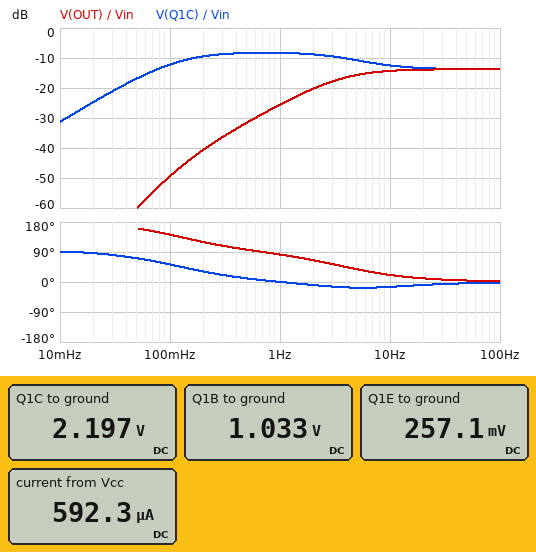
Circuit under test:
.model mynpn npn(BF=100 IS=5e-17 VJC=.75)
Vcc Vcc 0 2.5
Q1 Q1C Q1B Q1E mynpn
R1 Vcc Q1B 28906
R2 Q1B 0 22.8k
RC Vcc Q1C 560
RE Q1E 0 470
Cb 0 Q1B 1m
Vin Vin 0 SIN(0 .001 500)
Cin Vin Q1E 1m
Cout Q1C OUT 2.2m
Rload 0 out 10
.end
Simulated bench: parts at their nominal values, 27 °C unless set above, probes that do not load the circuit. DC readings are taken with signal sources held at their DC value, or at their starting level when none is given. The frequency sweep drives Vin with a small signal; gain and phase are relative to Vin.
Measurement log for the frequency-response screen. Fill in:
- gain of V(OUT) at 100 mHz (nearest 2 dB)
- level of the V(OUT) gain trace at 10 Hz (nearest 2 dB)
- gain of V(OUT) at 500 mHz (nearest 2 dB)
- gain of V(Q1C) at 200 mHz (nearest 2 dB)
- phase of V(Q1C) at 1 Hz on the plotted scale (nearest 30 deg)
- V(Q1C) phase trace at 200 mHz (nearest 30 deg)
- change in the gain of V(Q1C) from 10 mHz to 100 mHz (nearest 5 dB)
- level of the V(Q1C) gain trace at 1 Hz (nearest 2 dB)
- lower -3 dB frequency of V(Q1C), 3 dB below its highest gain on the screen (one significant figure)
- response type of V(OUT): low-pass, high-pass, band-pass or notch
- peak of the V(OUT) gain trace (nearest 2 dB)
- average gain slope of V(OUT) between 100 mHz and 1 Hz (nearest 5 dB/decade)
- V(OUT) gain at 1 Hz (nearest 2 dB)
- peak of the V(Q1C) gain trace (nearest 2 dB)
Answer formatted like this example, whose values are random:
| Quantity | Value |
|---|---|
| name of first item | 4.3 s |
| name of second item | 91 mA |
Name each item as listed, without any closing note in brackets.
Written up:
| Quantity | Value |
|---|---|
| gain of V(OUT) at 100 mHz | -50 dB |
| level of the V(OUT) gain trace at 10 Hz | -14 dB |
| gain of V(OUT) at 500 mHz | -32 dB |
| gain of V(Q1C) at 200 mHz | -10 dB |
| phase of V(Q1C) at 1 Hz on the plotted scale | 0 deg |
| V(Q1C) phase trace at 200 mHz | 30 deg |
| change in the gain of V(Q1C) from 10 mHz to 100 mHz | 20 dB |
| level of the V(Q1C) gain trace at 1 Hz | -8 dB |
| lower -3 dB frequency of V(Q1C), 3 dB below its highest gain on the screen | 100 mHz |
| response type of V(OUT): low-pass, high-pass, band-pass or notch | high-pass |
| peak of the V(OUT) gain trace | -14 dB |
| average gain slope of V(OUT) between 100 mHz and 1 Hz | 25 dB/decade |
| V(OUT) gain at 1 Hz | -26 dB |
| peak of the V(Q1C) gain trace | -8 dB |
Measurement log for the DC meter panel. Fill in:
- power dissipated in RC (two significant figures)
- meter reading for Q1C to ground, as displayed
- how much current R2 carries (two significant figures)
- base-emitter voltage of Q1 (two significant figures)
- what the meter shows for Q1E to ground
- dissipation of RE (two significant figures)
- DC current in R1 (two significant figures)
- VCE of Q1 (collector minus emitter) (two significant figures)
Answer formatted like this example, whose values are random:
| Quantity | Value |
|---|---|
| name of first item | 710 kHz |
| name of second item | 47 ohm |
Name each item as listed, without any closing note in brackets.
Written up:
| Quantity | Value |
|---|---|
| power dissipated in RC | 160 µW |
| meter reading for Q1C to ground, as displayed | 2.197 V |
| how much current R2 carries | 45 µA |
| base-emitter voltage of Q1 | 780 mV |
| what the meter shows for Q1E to ground | 257.1 mV |
| dissipation of RE | 140 µW |
| DC current in R1 | 51 µA |
| VCE of Q1 (collector minus emitter) | 1.9 V |
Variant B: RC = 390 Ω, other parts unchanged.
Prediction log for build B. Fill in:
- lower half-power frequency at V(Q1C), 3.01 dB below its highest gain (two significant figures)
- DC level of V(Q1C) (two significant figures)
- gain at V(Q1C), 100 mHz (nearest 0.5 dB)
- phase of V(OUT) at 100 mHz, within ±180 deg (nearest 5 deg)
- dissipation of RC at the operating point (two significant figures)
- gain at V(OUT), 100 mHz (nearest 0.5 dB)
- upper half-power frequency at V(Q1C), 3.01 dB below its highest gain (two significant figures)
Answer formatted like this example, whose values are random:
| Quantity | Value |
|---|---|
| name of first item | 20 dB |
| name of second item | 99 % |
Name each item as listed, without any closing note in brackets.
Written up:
| Quantity | Value |
|---|---|
| lower half-power frequency at V(Q1C), 3.01 dB below its highest gain | 170 mHz |
| DC level of V(Q1C) | 2.3 V |
| gain at V(Q1C), 100 mHz | -14.5 dB |
| phase of V(OUT) at 100 mHz, within ±180 deg | 150 deg |
| dissipation of RC at the operating point | 110 µW |
| gain at V(OUT), 100 mHz | -51.5 dB |
| upper half-power frequency at V(Q1C), 3.01 dB below its highest gain | 6.2 Hz |
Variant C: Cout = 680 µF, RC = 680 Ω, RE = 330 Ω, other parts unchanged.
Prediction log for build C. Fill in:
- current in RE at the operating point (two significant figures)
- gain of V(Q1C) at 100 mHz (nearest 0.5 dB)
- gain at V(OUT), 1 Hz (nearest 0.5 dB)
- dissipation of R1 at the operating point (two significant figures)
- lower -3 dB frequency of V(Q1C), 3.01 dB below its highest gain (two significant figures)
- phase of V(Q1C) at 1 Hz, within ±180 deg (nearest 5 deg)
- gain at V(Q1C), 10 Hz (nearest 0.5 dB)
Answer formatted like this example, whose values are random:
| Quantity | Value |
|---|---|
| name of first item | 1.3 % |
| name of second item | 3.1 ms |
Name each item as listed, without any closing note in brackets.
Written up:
| Quantity | Value |
|---|---|
| current in RE at the operating point | 700 µA |
| gain of V(Q1C) at 100 mHz | -9.0 dB |
| gain at V(OUT), 1 Hz | -26.0 dB |
| dissipation of R1 at the operating point | 76 µW |
| lower -3 dB frequency of V(Q1C), 3.01 dB below its highest gain | 300 mHz |
| phase of V(Q1C) at 1 Hz, within ±180 deg | 10 deg |
| gain at V(Q1C), 10 Hz | -4.5 dB |
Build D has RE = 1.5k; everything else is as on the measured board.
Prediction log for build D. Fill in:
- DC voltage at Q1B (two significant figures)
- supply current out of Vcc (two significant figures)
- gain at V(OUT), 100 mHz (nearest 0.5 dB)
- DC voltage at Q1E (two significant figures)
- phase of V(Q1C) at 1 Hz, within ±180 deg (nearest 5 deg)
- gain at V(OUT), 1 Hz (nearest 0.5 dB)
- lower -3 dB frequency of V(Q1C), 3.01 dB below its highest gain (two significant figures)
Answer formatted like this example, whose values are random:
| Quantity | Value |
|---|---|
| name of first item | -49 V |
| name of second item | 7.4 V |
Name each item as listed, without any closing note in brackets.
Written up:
| Quantity | Value |
|---|---|
| DC voltage at Q1B | 1.1 V |
| supply current out of Vcc | 260 µA |
| gain at V(OUT), 100 mHz | -49.0 dB |
| DC voltage at Q1E | 320 mV |
| phase of V(Q1C) at 1 Hz, within ±180 deg | -20 deg |
| gain at V(OUT), 1 Hz | -27.0 dB |
| lower -3 dB frequency of V(Q1C), 3.01 dB below its highest gain | 110 mHz |
